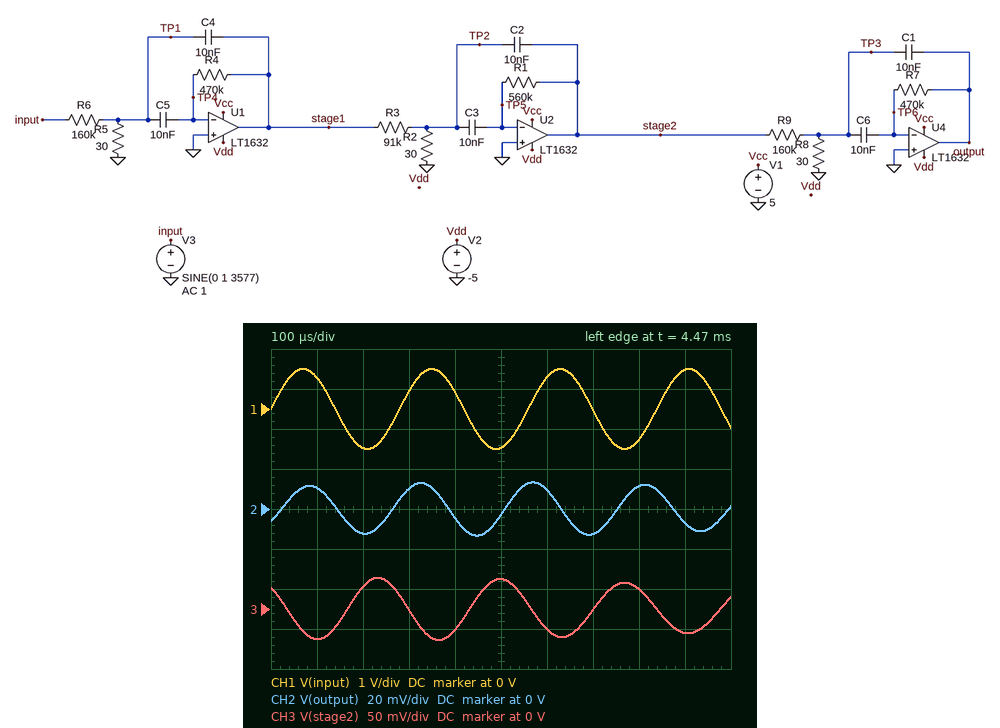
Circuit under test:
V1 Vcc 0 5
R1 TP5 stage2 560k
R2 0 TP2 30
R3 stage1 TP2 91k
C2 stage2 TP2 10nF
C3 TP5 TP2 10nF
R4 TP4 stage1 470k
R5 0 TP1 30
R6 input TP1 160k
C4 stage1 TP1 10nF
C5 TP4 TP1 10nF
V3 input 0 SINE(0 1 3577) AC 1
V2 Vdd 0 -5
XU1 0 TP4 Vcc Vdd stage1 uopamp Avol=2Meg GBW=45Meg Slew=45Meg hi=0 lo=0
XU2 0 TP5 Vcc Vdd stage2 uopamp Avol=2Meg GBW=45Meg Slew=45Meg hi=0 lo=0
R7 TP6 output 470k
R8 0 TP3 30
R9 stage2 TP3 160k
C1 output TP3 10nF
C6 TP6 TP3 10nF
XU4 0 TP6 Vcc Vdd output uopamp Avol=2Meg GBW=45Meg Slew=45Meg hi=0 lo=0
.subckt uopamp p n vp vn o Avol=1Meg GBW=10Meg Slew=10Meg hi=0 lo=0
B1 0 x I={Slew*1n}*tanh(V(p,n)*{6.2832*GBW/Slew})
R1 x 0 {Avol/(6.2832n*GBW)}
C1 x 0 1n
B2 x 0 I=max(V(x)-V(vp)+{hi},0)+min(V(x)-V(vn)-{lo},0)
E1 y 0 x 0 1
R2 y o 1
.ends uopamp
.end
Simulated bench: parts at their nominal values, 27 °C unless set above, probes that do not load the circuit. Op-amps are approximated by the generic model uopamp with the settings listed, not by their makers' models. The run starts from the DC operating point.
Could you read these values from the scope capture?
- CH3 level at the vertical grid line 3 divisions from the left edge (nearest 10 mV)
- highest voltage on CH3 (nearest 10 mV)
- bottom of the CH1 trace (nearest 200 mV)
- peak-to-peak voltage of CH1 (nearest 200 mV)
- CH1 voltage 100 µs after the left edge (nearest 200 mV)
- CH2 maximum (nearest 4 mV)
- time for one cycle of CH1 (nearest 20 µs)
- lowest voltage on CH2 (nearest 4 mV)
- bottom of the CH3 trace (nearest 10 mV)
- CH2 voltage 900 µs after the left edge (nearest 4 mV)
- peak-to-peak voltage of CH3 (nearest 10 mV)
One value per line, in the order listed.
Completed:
0 V
40 mV
-1.0 V
2.0 V
800 mV
12 mV
280 µs
-12 mV
-40 mV
-8 mV
80 mV
